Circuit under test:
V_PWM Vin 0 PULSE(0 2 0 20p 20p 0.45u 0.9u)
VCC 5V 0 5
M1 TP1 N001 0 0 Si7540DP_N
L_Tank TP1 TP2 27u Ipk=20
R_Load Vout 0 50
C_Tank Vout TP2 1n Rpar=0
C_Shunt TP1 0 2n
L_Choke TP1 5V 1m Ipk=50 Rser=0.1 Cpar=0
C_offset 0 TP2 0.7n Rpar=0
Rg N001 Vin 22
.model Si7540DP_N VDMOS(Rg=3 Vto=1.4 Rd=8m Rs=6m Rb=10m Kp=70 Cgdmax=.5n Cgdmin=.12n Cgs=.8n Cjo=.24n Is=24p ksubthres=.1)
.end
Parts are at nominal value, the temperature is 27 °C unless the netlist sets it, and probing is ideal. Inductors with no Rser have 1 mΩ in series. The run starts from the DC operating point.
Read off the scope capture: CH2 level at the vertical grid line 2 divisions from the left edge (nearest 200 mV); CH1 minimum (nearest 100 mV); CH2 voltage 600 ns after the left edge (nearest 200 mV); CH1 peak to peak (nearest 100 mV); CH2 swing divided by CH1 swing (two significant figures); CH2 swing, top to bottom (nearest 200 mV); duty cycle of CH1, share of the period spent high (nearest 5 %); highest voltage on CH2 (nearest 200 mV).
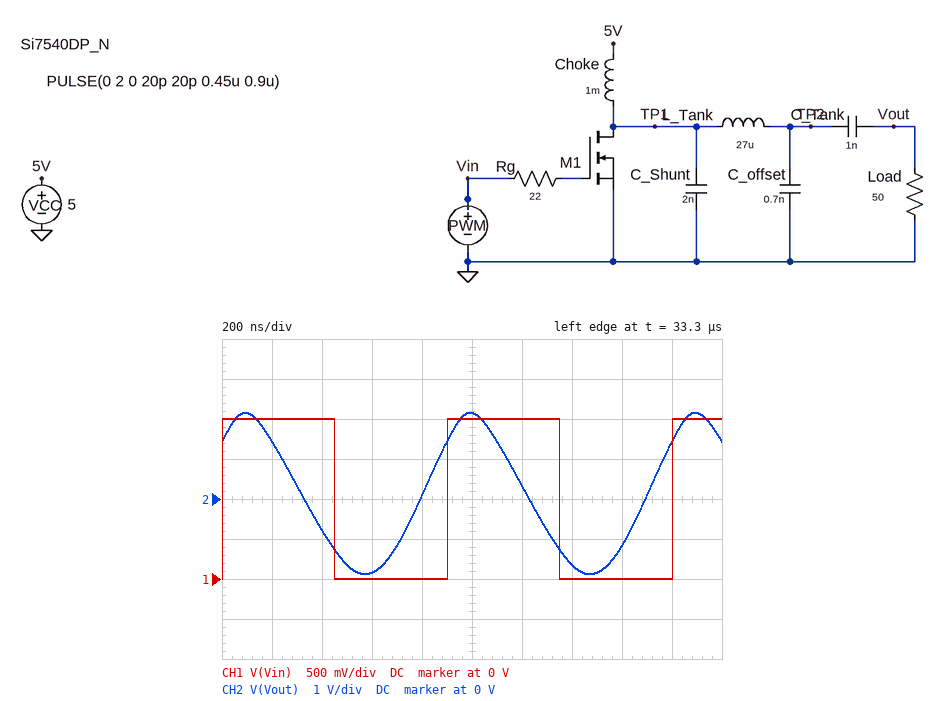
-800 mV
0 V
-1.8 V
2.0 V
2.0
4.0 V
50 %
2.2 V
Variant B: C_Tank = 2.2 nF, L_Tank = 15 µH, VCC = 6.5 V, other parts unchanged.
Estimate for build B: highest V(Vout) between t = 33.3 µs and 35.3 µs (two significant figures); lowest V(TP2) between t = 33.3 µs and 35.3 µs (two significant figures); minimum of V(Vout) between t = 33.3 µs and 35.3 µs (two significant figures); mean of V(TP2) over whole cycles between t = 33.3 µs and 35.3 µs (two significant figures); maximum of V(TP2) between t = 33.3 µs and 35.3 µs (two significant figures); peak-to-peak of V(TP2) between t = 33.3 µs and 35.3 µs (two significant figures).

5.9 V
-3.2 V
-5.5 V
6.4 V
16 V
19 V
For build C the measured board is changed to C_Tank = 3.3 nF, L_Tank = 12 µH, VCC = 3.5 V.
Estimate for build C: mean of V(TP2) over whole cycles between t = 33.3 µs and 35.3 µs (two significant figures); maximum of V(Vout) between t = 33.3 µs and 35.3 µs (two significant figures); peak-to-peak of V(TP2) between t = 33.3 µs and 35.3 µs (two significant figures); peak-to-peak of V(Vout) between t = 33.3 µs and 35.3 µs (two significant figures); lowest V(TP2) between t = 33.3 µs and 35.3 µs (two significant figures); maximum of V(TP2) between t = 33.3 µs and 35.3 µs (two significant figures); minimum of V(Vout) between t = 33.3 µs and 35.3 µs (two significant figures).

3.2 V
3.6 V
9.5 V
6.8 V
-1.4 V
8.1 V
-3.2 V
